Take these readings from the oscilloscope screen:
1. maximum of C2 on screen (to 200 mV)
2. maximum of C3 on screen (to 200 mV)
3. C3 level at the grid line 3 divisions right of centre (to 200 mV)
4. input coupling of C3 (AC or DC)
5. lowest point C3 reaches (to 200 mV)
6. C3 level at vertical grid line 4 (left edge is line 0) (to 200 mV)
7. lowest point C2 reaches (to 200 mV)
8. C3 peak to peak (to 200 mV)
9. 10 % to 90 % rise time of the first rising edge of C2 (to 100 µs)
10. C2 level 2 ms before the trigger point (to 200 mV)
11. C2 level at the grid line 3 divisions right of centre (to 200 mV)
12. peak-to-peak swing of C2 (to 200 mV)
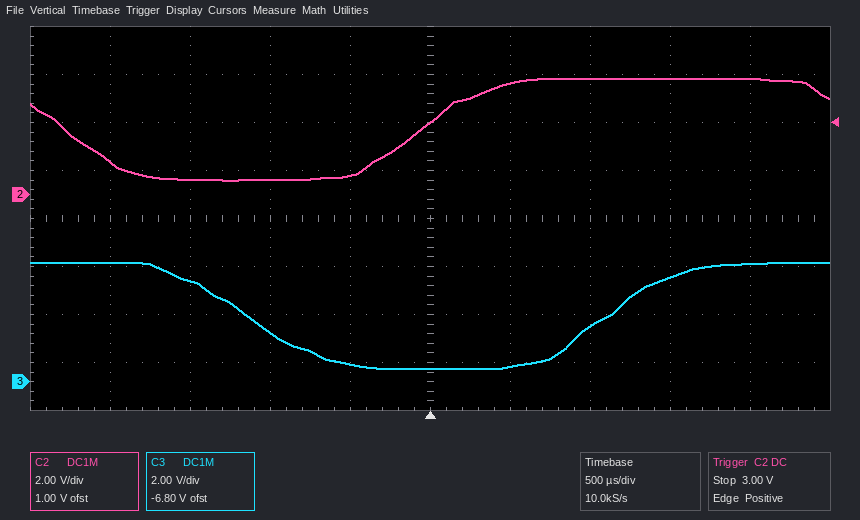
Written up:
4.8 V
5.0 V
4.4 V
DC
600 mV
800 mV
600 mV
4.4 V
800 µs
1.4 V
4.8 V
4.2 V
